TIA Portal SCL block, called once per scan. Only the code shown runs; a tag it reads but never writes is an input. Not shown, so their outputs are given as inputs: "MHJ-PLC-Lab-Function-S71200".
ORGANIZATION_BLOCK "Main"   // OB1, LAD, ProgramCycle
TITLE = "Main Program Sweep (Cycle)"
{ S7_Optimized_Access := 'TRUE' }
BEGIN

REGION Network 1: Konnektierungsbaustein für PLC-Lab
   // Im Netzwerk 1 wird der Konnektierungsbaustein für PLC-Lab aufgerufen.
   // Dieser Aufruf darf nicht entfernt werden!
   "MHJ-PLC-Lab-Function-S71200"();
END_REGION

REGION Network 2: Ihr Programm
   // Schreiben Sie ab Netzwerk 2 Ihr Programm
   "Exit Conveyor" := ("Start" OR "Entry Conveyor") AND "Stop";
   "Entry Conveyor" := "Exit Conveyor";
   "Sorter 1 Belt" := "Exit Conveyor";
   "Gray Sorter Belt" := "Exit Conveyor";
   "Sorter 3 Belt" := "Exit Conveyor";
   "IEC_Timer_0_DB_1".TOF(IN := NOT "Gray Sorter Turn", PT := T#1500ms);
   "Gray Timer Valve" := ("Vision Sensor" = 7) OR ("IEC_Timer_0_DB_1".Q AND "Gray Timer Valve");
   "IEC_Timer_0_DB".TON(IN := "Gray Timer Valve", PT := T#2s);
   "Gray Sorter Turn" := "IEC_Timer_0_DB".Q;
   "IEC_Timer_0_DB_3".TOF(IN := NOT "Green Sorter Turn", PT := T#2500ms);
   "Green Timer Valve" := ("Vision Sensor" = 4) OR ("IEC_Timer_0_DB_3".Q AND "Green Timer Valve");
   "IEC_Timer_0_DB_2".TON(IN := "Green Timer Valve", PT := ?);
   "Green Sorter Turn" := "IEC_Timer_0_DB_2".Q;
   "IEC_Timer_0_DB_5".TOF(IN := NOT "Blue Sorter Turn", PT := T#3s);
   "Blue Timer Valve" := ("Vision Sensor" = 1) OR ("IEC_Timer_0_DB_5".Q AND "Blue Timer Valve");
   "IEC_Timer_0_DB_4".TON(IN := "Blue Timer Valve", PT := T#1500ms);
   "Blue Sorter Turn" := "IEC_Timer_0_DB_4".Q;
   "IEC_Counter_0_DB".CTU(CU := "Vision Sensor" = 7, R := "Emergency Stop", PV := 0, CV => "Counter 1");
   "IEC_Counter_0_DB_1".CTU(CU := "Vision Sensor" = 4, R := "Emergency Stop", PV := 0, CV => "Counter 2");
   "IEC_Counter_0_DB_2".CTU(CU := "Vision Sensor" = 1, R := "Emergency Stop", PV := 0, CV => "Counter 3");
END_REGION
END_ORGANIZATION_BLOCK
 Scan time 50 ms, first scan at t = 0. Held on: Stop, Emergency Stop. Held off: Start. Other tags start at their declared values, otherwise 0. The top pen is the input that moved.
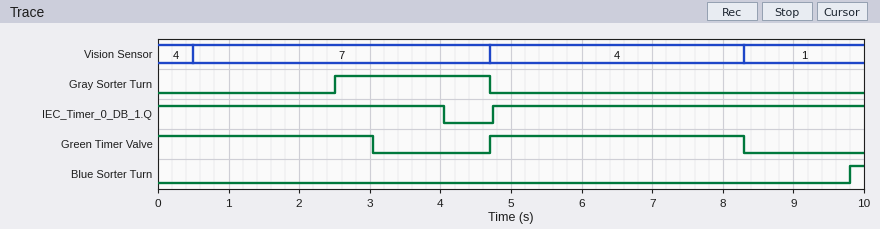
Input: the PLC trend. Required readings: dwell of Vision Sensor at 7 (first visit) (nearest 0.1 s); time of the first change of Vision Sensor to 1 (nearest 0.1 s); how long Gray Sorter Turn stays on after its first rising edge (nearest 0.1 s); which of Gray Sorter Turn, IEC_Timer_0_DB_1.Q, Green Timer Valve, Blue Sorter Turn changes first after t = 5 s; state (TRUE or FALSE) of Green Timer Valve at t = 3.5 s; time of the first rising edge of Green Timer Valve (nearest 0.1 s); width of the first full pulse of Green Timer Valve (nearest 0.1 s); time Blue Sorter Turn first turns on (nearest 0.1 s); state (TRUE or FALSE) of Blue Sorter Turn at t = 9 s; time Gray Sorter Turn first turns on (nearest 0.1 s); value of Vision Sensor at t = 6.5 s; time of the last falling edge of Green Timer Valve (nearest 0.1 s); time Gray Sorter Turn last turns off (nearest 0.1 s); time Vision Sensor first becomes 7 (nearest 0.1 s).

4.2 s
8.3 s
2.2 s
Green Timer Valve
FALSE
4.7 s
3.6 s
9.8 s
FALSE
2.5 s
4
8.3 s
4.7 s
0.5 s
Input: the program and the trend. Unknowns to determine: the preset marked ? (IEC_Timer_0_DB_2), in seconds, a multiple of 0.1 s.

0.5 s
